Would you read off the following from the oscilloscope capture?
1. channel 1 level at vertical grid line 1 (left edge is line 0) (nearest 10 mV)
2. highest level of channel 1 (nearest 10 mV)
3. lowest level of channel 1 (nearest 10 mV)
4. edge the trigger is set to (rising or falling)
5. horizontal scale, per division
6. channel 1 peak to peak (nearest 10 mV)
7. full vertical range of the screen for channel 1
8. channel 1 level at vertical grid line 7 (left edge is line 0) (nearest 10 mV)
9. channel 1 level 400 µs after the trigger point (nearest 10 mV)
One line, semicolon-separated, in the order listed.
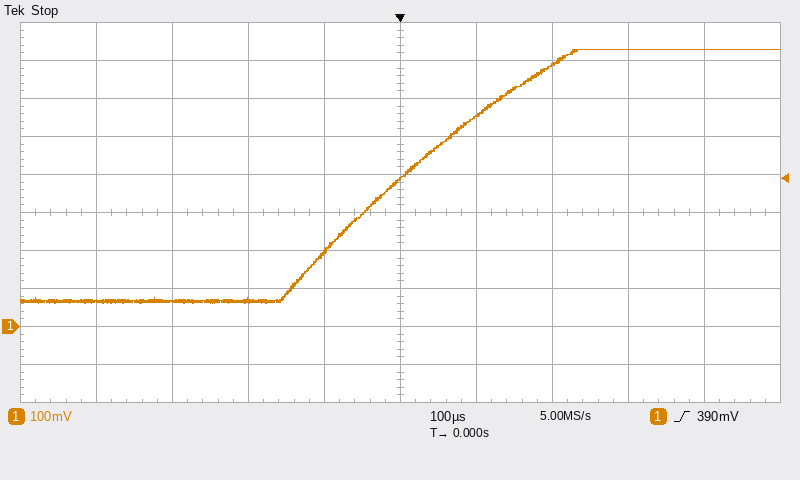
70 mV; 730 mV; 60 mV; rising; 100 µs; 670 mV; 1 V; 690 mV; 730 mV
